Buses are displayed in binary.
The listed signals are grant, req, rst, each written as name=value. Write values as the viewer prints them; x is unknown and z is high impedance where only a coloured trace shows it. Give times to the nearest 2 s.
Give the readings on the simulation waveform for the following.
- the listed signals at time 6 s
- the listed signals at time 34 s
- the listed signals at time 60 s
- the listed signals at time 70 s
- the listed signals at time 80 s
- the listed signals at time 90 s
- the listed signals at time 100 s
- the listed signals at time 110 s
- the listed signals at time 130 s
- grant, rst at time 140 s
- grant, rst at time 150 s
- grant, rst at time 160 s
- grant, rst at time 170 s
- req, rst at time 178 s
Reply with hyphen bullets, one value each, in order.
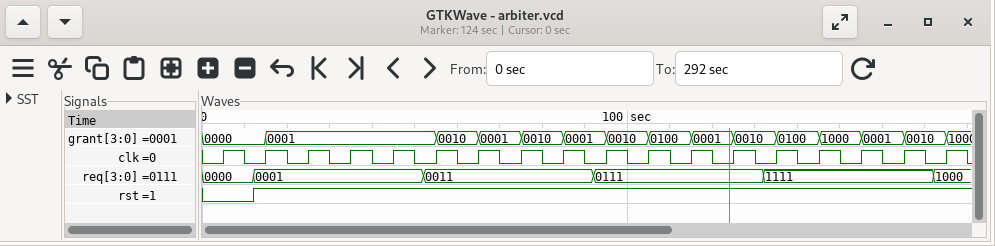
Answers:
- grant=0000, req=0000, rst=0
- grant=0001, req=0001, rst=1
- grant=0010, req=0011, rst=1
- grant=0001, req=0011, rst=1
- grant=0010, req=0011, rst=1
- grant=0001, req=0011, rst=1
- grant=0010, req=0111, rst=1
- grant=0100, req=0111, rst=1
- grant=0010, req=0111, rst=1
- grant=0100, rst=1
- grant=1000, rst=1
- grant=0001, rst=1
- grant=0010, rst=1
- req=1000, rst=1
